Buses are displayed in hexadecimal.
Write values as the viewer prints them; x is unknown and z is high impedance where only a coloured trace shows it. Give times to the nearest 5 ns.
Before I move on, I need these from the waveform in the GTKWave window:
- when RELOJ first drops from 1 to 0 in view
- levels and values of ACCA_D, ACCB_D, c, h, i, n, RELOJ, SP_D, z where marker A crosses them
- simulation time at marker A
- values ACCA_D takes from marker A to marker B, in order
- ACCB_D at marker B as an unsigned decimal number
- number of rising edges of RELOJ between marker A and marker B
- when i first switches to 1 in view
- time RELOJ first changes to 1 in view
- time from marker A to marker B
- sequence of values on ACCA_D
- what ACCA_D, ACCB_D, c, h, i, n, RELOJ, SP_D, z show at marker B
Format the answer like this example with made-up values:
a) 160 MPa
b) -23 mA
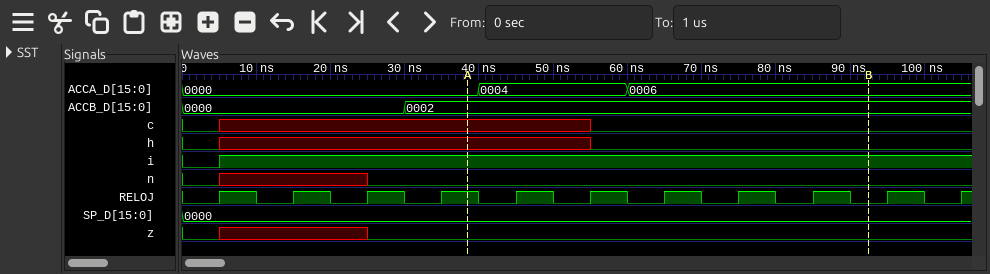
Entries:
a) 10 ns
b) ACCA_D=0000, ACCB_D=0002, c=x, h=x, i=1, n=0, RELOJ=1, SP_D=0000, z=0
c) 40 ns
d) 0000, 0004, 0006
e) 2
f) 5
g) 5 ns
h) 5 ns
i) 55 ns
j) 0000, 0004, 0006
k) ACCA_D=0006, ACCB_D=0002, c=0, h=0, i=1, n=0, RELOJ=0, SP_D=0000, z=0
